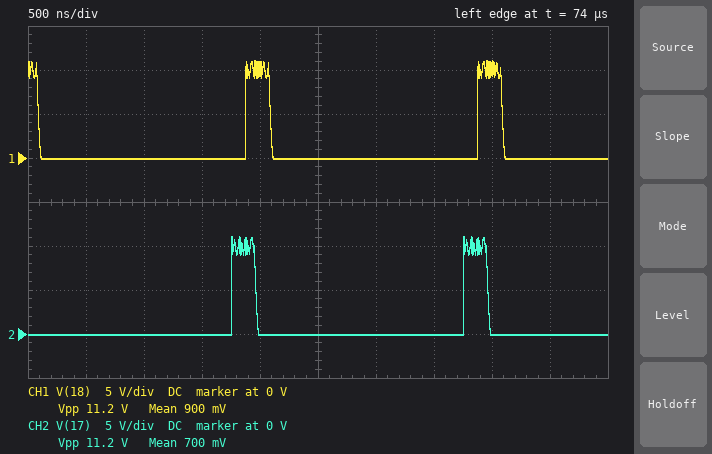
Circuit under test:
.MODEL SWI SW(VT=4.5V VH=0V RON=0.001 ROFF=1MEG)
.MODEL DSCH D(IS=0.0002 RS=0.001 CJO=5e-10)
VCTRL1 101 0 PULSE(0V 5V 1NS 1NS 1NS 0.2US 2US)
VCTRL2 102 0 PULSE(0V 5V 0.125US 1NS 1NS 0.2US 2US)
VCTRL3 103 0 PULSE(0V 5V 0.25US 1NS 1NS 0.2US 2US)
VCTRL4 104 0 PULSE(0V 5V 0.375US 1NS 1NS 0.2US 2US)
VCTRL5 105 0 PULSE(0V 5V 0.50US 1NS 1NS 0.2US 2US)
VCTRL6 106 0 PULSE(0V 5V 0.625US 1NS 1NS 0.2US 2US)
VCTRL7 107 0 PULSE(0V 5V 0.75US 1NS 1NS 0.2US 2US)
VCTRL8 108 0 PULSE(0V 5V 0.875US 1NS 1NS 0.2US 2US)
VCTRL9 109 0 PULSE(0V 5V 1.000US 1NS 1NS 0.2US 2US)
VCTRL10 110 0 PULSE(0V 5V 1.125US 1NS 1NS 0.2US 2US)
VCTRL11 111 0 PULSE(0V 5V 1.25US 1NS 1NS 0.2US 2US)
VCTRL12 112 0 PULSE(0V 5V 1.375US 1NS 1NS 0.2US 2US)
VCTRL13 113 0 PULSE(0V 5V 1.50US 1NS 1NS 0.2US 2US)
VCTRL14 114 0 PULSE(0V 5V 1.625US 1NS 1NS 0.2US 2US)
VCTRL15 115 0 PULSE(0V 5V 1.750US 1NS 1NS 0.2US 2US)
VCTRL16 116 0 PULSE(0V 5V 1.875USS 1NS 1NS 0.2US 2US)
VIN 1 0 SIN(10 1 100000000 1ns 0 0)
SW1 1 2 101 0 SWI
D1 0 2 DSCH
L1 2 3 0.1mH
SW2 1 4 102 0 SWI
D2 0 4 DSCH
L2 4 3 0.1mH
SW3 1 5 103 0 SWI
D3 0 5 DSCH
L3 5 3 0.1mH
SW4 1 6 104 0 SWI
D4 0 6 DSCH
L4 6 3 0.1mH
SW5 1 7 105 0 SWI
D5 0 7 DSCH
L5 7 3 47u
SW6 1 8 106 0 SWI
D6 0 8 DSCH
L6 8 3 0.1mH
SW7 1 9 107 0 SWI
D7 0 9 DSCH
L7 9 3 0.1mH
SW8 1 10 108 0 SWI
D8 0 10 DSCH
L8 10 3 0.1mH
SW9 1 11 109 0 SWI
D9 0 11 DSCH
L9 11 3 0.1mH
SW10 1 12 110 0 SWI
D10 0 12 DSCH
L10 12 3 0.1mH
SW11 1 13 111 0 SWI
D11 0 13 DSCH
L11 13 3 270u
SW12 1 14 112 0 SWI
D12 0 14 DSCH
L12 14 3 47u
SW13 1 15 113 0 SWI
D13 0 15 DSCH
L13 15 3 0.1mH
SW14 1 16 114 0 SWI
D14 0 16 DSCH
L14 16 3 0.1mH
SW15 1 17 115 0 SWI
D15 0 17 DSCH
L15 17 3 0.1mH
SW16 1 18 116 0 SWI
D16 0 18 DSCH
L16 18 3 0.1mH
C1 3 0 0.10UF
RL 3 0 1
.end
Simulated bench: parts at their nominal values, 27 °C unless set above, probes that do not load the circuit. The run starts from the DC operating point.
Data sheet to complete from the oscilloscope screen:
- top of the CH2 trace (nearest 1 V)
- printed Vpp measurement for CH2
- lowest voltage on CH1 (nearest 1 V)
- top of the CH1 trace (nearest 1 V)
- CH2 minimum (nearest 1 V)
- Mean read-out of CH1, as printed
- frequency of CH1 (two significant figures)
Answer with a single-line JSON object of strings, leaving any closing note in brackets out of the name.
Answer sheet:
{"top of the CH2 trace": "11 V", "printed Vpp measurement for CH2": "11.2 V", "lowest voltage on CH1": "0 V", "top of the CH1 trace": "11 V", "CH2 minimum": "0 V", "Mean read-out of CH1, as printed": "900 mV", "frequency of CH1": "500 kHz"}
